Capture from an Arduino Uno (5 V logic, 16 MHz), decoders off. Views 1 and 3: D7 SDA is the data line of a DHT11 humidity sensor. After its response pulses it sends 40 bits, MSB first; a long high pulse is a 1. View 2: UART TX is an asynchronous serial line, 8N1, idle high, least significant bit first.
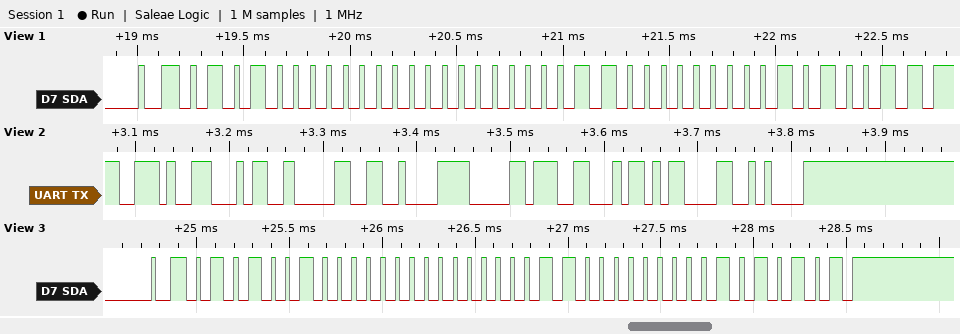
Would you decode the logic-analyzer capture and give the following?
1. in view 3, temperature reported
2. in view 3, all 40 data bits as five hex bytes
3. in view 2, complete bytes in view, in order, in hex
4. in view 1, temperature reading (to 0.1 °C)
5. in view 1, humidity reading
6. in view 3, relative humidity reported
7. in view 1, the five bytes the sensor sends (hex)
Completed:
3.0 °C
52 00 03 00 55
2E 34 30 C2 B0 46 0D 0A
3.0 °C
80 %
82 %
50 00 03 00 53
